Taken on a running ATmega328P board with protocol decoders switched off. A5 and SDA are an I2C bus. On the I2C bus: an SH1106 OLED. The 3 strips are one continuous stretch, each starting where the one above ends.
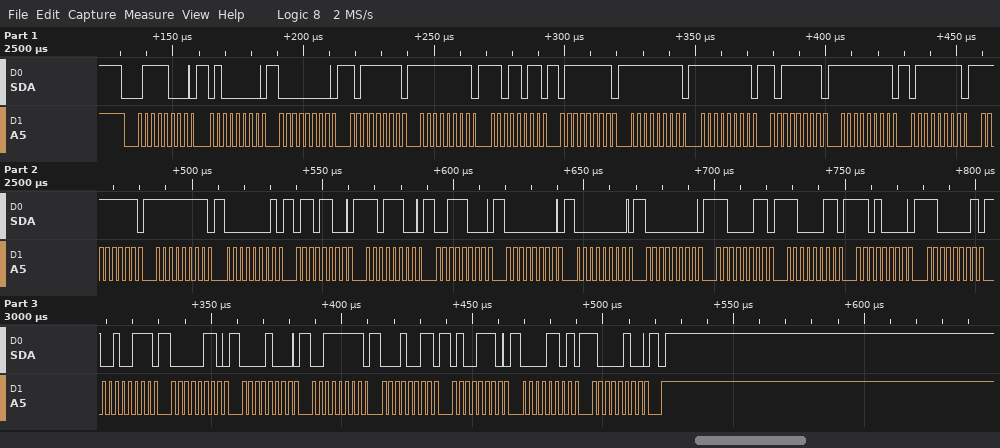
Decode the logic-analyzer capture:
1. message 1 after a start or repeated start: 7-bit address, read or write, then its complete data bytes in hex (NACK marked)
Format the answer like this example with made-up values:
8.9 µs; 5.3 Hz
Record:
0x3C write: 40 00 BF FF DB 7F FF FF BF FF 7F FF FF 01 6C DC 38 00 00 00 C3 C3 D0 C1 27 06 08 3F 13 4E 0D 84
